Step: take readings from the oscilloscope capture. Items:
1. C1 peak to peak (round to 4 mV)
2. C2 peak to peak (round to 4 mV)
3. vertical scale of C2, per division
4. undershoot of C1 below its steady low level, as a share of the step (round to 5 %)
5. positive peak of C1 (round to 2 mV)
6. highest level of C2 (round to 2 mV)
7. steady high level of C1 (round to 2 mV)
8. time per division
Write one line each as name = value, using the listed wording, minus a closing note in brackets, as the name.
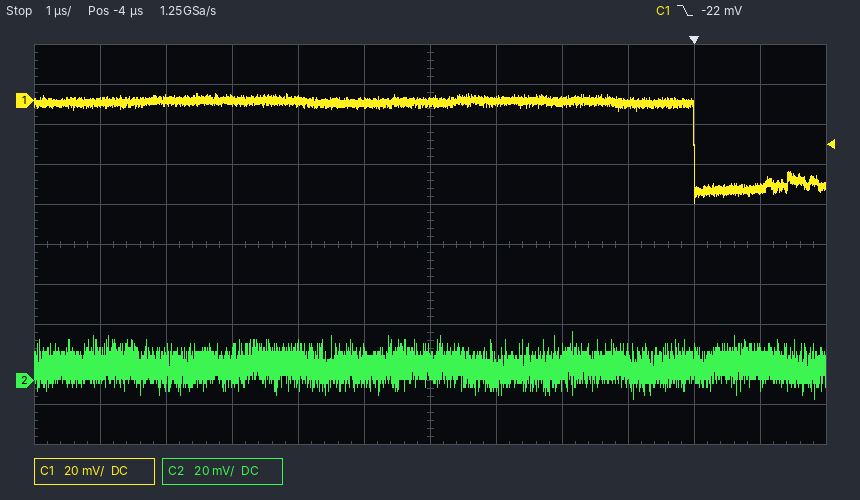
C1 peak to peak = 56 mV
C2 peak to peak = 32 mV
vertical scale of C2, per division = 20 mV
undershoot of C1 below its steady low level, as a share of the step = 15 %
positive peak of C1 = 4 mV
highest level of C2 = 24 mV
steady high level of C1 = 0 mV
time per division = 1 µs
